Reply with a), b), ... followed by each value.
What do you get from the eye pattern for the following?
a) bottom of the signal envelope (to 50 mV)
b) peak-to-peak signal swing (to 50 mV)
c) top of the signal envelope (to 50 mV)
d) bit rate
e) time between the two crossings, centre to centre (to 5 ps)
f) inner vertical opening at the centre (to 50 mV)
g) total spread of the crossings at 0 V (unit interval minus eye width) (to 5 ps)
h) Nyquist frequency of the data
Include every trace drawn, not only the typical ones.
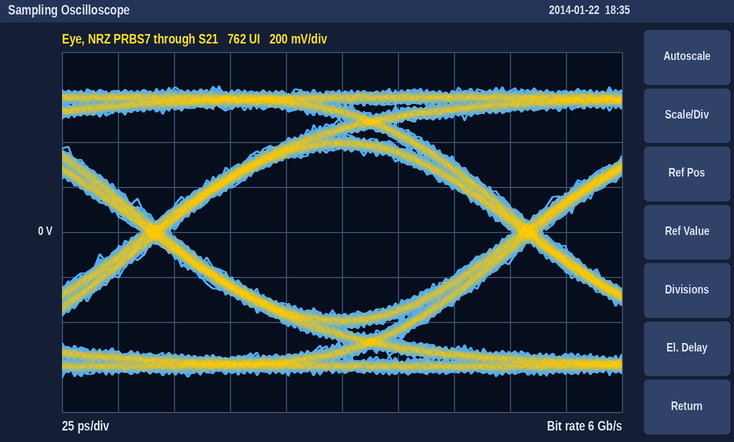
a) -650 mV
b) 1.30 V
c) 650 mV
d) 6 Gb/s
e) 165 ps
f) 750 mV
g) 15 ps
h) 3 GHz
